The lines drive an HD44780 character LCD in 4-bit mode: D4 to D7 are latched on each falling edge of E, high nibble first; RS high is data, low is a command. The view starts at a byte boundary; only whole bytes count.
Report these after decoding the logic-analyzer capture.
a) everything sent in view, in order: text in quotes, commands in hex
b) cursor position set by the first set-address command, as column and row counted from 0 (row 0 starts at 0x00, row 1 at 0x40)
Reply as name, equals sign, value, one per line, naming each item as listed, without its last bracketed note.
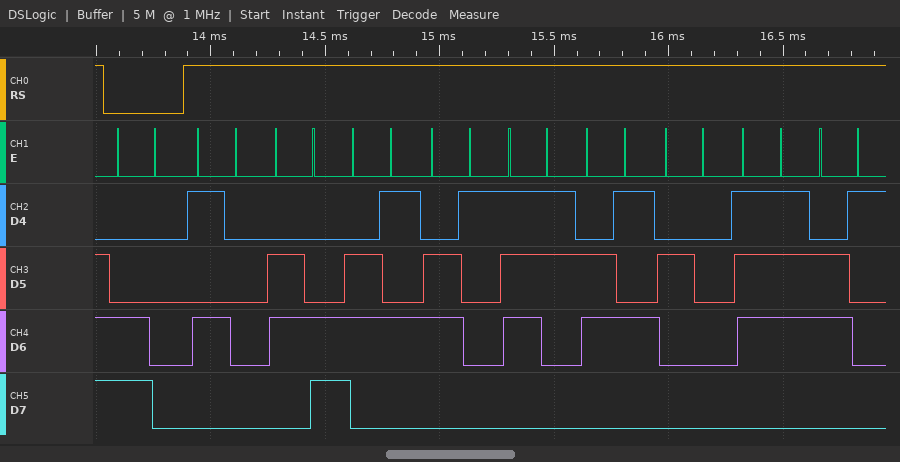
everything sent in view, in order: text in quotes, commands in hex = 0xC0 "Please wa"
cursor position set by the first set-address command, as column and row counted from 0 = column 0, row 1
